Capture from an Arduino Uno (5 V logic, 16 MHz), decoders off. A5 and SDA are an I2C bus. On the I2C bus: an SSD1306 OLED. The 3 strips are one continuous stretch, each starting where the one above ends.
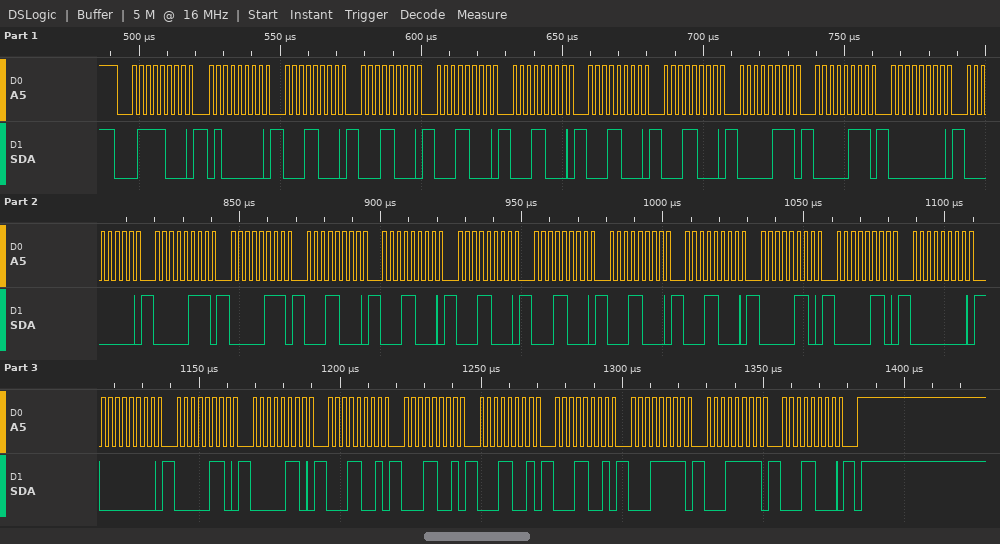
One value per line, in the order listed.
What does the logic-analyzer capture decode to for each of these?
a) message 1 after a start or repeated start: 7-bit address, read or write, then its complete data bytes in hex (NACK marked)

0x3C write: 40 18 18 18 18 18 18 07 07 00 00 07 07 18 18 18 18 18 18 06 06 00 00 06 06 19 19 19 19 1F 1F 18
